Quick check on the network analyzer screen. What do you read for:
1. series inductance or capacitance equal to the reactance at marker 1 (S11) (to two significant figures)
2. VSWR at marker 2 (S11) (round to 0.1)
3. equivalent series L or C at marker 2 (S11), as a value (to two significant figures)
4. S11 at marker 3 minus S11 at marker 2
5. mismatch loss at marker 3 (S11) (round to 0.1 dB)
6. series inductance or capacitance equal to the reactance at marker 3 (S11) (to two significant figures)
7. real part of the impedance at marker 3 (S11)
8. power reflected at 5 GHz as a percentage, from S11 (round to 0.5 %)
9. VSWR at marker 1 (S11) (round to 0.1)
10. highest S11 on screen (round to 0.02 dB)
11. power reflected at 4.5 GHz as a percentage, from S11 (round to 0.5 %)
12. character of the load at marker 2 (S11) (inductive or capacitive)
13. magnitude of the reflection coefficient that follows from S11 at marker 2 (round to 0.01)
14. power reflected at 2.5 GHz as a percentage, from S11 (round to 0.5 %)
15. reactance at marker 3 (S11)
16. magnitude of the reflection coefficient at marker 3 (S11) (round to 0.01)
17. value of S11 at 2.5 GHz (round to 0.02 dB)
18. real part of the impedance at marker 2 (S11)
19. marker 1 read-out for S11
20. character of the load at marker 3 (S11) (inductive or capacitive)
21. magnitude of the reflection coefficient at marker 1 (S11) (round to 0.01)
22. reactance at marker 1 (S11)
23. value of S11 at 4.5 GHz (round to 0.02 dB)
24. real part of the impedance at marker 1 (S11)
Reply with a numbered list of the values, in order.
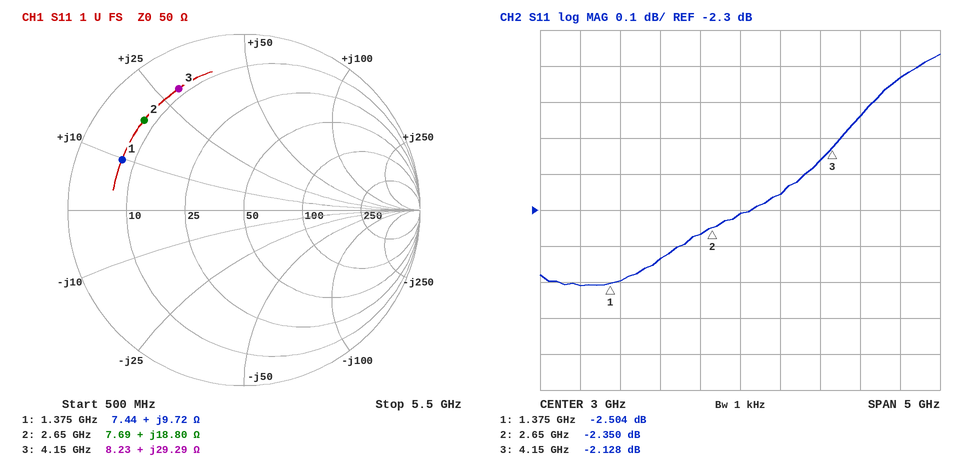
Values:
1. 1.1 nH
2. 7.4
3. 1.1 nH
4. 0.222 dB
5. 4.1 dB
6. 1.1 nH
7. 8.23 Ω
8. 64.0 %
9. 7.0
10. -1.86 dB
11. 62.5 %
12. inductive
13. 0.76
14. 58.0 %
15. +29.29 Ω
16. 0.78
17. -2.36 dB
18. 7.69 Ω
19. -2.504 dB
20. inductive
21. 0.75
22. +9.72 Ω
23. -2.04 dB
24. 7.44 Ω
